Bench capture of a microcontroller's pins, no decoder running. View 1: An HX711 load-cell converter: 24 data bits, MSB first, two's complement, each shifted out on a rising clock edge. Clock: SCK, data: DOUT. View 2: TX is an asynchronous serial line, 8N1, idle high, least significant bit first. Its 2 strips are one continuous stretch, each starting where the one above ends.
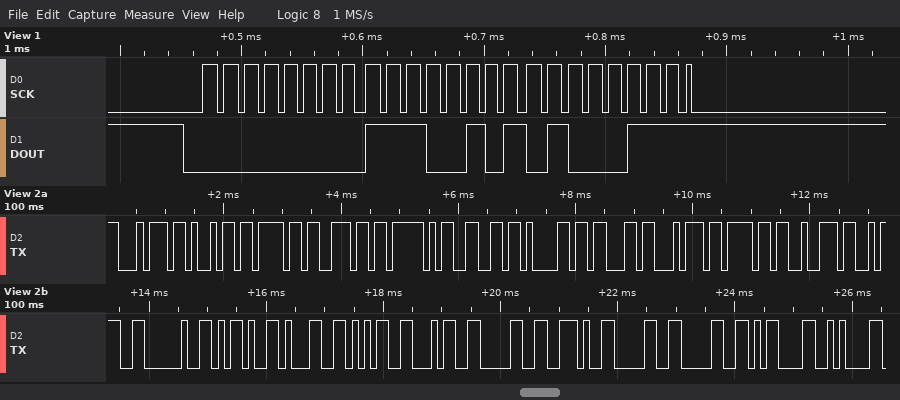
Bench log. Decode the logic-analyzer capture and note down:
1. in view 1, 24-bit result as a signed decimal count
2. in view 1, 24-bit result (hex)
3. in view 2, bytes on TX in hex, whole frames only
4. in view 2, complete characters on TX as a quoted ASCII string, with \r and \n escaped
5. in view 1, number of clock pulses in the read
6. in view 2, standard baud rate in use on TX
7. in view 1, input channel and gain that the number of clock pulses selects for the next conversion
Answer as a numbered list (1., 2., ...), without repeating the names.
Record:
1. 58695
2. 0x00E547
3. 74 69 6F 6E 5F 66 61 63 74 6F 72 3A 20 2D 31 35 34 30 2E 30 30 0D 0A
4. "tion_factor: -1540.00\r\n"
5. 25
6. 9600 baud
7. channel A, gain 128
